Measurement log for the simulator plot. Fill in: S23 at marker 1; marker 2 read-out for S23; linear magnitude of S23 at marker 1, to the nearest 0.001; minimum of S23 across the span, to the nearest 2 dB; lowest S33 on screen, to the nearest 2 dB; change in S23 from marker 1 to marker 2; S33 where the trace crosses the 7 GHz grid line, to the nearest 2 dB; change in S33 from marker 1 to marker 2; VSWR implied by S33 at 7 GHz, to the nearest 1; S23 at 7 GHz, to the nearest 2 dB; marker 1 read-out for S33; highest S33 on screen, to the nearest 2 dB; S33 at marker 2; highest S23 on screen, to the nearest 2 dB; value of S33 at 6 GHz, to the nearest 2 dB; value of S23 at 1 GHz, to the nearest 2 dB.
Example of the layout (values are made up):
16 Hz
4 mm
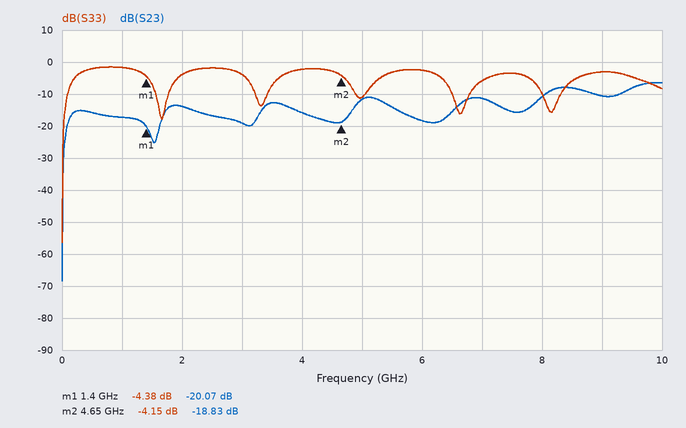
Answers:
-20.07 dB
-18.83 dB
0.099
-68 dB
-56 dB
1.24 dB
-6 dB
0.23 dB
3
-12 dB
-4.38 dB
-2 dB
-4.15 dB
-6 dB
-2 dB
-18 dB
